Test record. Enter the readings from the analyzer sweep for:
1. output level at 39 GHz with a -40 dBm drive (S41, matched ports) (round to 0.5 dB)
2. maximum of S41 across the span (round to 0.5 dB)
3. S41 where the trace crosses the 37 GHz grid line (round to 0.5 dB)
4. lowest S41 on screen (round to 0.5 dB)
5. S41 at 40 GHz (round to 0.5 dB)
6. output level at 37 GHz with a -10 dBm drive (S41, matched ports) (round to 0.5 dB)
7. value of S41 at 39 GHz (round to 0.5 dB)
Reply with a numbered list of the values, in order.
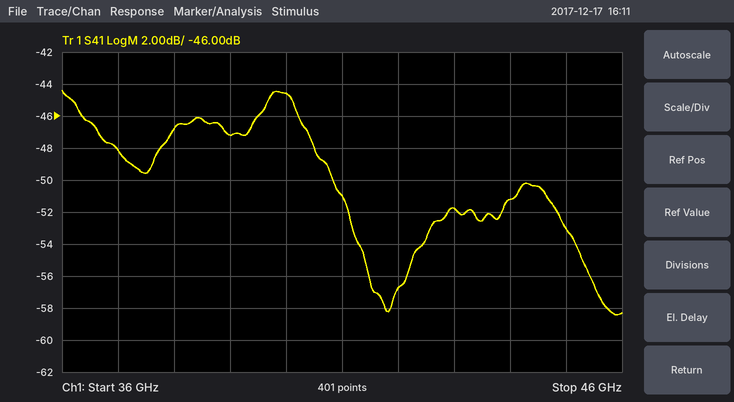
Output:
1. -87.0 dBm
2. -44.5 dB
3. -48.0 dB
4. -58.5 dB
5. -44.5 dB
6. -58.0 dBm
7. -47.0 dB
